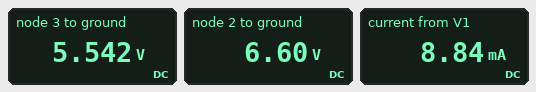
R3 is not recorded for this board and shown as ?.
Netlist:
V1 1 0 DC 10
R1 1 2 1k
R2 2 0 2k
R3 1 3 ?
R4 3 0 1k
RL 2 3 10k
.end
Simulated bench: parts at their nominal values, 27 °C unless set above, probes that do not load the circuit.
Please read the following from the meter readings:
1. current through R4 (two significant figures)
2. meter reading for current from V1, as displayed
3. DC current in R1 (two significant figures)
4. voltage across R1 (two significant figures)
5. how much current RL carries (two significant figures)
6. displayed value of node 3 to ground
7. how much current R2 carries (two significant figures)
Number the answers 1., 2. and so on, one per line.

1. 5.5 mA
2. 8.84 mA
3. 3.4 mA
4. 3.4 V
5. 110 µA
6. 5.542 V
7. 3.3 mA
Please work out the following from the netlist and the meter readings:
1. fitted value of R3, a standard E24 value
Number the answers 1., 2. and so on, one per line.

1. 820 Ω
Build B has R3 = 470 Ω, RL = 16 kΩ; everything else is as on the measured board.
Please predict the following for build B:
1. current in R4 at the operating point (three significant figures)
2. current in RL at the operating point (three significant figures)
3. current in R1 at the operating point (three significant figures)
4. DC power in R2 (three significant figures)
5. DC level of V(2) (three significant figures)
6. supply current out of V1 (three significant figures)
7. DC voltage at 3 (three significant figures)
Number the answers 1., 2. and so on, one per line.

1. 6.80 mA
2. 8.01 µA
3. 3.33 mA
4. 22.3 mW
5. 6.67 V
6. 10.1 mA
7. 6.80 V
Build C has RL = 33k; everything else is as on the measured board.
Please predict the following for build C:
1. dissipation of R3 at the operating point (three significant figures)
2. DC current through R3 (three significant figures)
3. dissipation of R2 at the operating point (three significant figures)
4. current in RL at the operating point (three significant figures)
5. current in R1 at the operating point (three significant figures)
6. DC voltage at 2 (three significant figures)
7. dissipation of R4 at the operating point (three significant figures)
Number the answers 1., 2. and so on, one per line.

1. 24.6 mW
2. 5.48 mA
3. 22.1 mW
4. 34.4 µA
5. 3.36 mA
6. 6.64 V
7. 30.4 mW
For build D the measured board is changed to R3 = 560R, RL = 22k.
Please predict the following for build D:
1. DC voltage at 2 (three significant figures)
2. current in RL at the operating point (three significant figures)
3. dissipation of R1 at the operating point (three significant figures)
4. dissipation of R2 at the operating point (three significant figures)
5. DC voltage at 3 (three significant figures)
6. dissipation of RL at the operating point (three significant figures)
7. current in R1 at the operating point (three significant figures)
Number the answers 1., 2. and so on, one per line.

1. 6.66 V
2. 11.1 µA
3. 11.2 mW
4. 22.2 mW
5. 6.41 V
6. 2.73 µW
7. 3.34 mA
